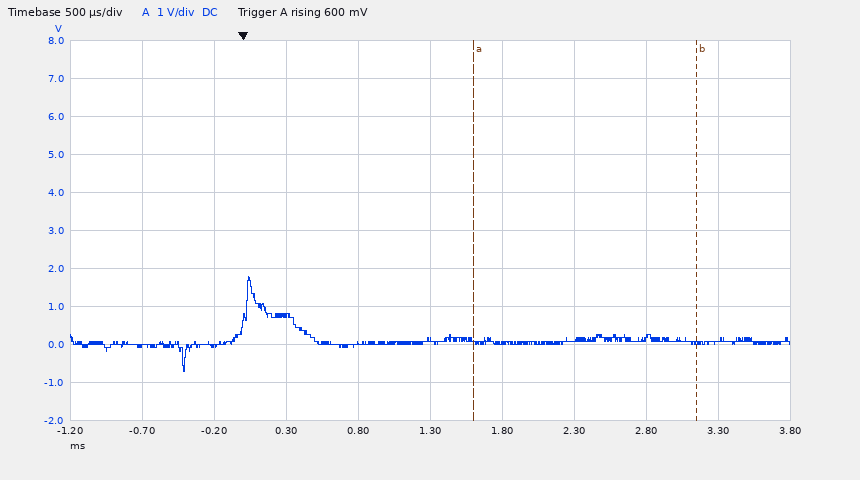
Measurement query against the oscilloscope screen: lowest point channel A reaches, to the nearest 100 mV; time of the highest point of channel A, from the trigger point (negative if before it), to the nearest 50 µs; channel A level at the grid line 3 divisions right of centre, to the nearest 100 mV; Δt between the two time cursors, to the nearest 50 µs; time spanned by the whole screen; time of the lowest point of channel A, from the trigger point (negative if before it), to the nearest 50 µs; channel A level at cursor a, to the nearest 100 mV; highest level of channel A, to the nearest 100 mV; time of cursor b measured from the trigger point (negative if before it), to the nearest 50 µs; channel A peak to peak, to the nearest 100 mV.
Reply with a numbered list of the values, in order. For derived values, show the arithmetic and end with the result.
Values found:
1. -700 mV
2. +50 µs
3. 200 mV
4. 1.55 ms
5. 5 ms
6. -400 µs
7. 100 mV
8. 1.8 V
9. +3.15 ms
10. 1.8 V − (-700 mV) = 2.5 V
